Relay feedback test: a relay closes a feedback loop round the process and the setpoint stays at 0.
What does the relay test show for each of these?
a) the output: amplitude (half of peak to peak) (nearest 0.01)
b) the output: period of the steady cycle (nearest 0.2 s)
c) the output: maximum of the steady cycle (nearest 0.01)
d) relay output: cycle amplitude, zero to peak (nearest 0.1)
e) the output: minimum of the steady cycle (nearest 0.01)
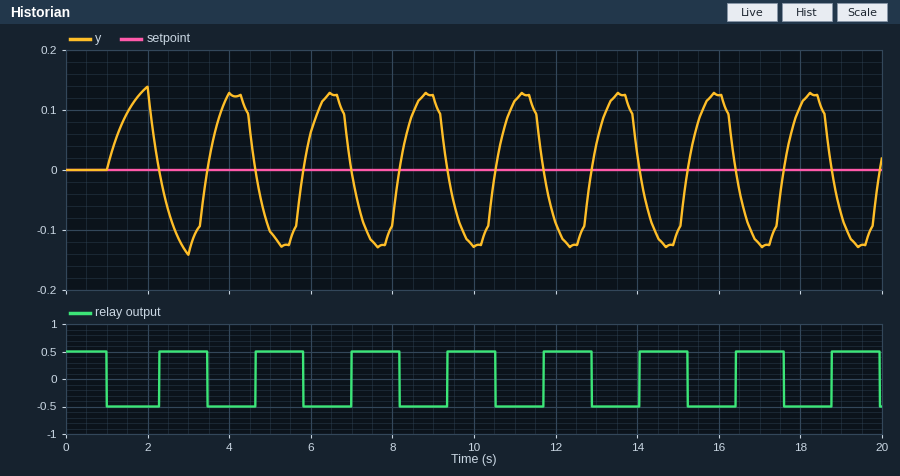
0.13
2.4 s
0.13
0.5
-0.13
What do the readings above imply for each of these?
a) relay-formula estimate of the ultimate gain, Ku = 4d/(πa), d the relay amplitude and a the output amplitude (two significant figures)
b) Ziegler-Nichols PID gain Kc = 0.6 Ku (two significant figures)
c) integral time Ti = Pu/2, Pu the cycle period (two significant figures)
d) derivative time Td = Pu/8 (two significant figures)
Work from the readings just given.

4.9
2.9
1.2 s
0.30 s
